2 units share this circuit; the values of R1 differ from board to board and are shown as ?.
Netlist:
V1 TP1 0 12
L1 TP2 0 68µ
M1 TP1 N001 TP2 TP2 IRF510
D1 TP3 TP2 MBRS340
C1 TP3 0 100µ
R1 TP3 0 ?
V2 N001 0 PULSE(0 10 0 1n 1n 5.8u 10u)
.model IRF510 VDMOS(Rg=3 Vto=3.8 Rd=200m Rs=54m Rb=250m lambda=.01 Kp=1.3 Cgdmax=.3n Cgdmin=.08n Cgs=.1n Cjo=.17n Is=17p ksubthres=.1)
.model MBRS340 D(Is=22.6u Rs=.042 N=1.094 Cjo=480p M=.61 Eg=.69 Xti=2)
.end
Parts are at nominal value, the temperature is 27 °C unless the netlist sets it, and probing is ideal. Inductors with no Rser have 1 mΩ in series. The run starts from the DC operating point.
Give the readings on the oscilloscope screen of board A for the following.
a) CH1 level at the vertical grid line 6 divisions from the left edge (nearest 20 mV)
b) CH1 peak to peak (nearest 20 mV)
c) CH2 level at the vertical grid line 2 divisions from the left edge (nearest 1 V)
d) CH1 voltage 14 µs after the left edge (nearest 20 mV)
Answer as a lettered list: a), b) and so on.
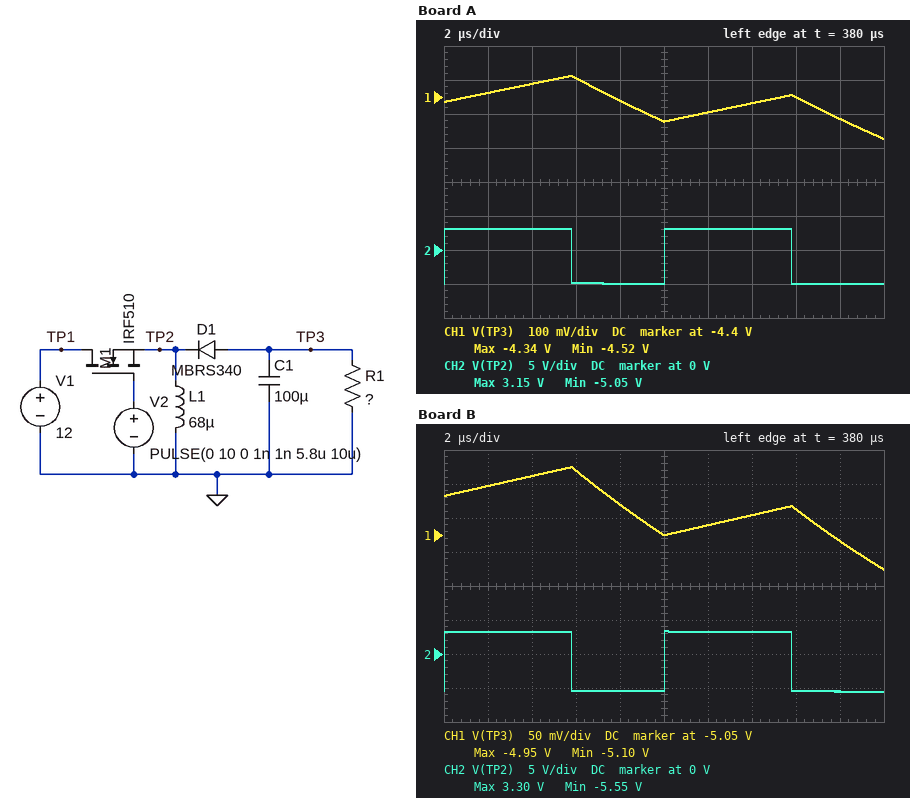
a) -4.44 V
b) 180 mV
c) 3 V
d) -4.42 V
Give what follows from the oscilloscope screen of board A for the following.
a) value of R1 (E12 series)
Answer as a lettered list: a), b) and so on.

a) 3.3 Ω
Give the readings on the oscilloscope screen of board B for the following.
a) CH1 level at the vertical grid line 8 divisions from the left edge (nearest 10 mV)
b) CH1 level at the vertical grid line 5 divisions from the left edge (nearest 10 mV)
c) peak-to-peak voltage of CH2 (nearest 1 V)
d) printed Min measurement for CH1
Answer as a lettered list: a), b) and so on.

a) -5.01 V
b) -5.05 V
c) 9 V
d) -5.10 V
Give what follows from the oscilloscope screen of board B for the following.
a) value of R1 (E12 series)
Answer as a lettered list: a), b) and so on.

a) 6.8 Ω
